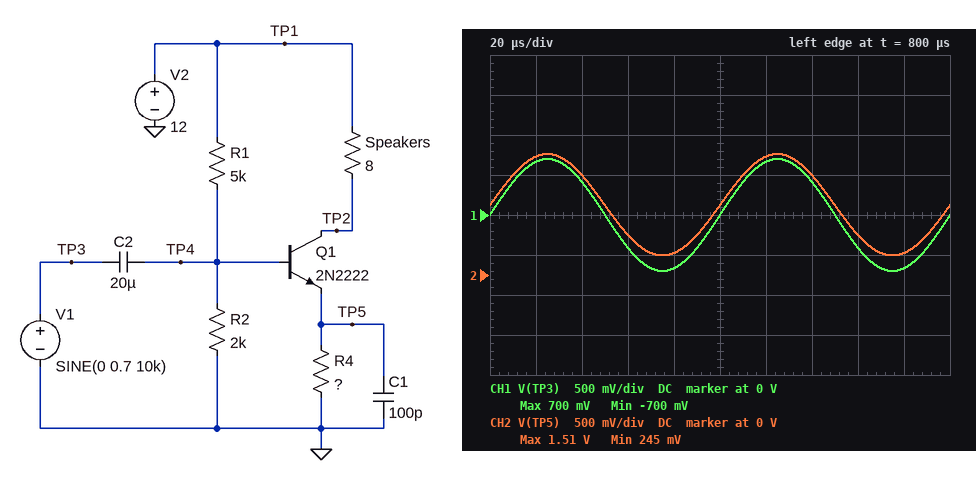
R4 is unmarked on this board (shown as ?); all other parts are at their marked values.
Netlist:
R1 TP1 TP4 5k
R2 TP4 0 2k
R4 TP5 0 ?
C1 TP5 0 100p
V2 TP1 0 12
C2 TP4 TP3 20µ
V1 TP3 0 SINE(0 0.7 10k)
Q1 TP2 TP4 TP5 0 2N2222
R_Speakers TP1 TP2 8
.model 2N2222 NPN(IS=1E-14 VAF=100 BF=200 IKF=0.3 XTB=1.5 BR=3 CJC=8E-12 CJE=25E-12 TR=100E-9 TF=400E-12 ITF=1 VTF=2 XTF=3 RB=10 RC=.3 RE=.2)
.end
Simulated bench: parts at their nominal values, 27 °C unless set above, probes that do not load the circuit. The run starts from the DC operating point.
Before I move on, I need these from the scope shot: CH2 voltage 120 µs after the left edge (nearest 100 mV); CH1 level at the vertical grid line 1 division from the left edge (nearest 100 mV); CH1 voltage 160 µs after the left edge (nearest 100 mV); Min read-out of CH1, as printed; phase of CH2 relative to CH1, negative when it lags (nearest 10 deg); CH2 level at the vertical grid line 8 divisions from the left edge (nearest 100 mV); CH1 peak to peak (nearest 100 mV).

1.5 V
700 mV
-400 mV
-700 mV
0 deg
500 mV
1.4 V
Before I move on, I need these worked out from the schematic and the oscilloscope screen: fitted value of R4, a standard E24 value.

5.1 Ω
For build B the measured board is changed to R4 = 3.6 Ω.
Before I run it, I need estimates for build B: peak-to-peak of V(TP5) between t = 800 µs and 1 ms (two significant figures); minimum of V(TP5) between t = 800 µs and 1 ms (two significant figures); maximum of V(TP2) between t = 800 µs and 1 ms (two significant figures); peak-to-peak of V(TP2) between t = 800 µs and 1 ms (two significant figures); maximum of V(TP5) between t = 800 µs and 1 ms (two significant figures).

1.2 V
74 mV
12 V
2.7 V
1.3 V
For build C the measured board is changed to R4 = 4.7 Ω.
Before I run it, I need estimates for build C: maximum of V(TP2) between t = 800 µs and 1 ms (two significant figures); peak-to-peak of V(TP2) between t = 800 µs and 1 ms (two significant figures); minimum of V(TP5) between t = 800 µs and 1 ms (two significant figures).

12 V
2.1 V
200 mV
